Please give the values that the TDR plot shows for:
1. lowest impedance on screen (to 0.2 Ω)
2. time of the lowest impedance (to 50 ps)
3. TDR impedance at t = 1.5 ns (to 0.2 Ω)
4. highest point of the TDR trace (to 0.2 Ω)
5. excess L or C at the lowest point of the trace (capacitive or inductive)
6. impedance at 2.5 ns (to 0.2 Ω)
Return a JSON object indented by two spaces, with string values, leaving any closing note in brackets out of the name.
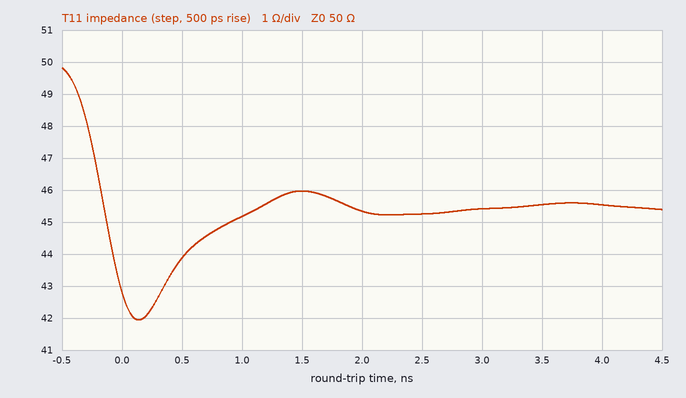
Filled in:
{
  "lowest impedance on screen": "42.0 Ω",
  "time of the lowest impedance": "150 ps",
  "TDR impedance at t = 1.5 ns": "46.0 Ω",
  "highest point of the TDR trace": "49.8 Ω",
  "excess L or C at the lowest point of the trace": "capacitive",
  "impedance at 2.5 ns": "45.2 Ω"
}
